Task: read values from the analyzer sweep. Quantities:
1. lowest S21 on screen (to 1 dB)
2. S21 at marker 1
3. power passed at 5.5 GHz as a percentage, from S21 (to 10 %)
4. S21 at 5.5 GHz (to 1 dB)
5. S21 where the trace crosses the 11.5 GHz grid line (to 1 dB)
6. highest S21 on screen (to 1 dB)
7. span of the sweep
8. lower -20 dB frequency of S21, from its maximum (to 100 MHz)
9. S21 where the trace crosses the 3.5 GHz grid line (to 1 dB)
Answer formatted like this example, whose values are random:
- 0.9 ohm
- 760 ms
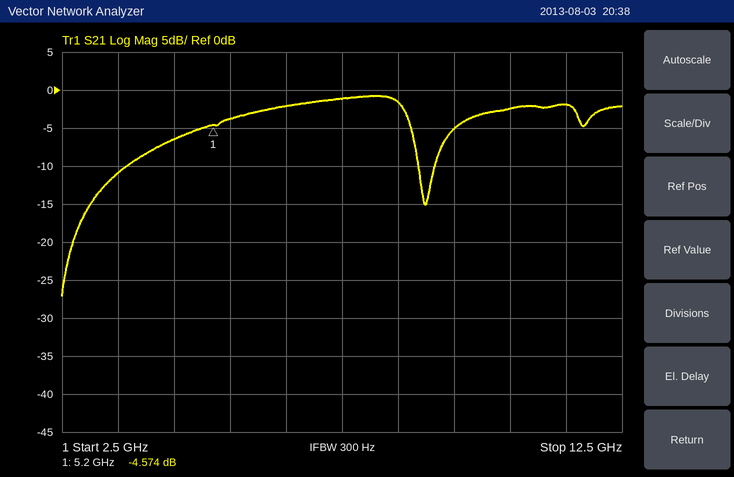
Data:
- -27 dB
- -4.574 dB
- 40 %
- -4 dB
- -2 dB
- -1 dB
- 10 GHz
- 2.7 GHz
- -11 dB
